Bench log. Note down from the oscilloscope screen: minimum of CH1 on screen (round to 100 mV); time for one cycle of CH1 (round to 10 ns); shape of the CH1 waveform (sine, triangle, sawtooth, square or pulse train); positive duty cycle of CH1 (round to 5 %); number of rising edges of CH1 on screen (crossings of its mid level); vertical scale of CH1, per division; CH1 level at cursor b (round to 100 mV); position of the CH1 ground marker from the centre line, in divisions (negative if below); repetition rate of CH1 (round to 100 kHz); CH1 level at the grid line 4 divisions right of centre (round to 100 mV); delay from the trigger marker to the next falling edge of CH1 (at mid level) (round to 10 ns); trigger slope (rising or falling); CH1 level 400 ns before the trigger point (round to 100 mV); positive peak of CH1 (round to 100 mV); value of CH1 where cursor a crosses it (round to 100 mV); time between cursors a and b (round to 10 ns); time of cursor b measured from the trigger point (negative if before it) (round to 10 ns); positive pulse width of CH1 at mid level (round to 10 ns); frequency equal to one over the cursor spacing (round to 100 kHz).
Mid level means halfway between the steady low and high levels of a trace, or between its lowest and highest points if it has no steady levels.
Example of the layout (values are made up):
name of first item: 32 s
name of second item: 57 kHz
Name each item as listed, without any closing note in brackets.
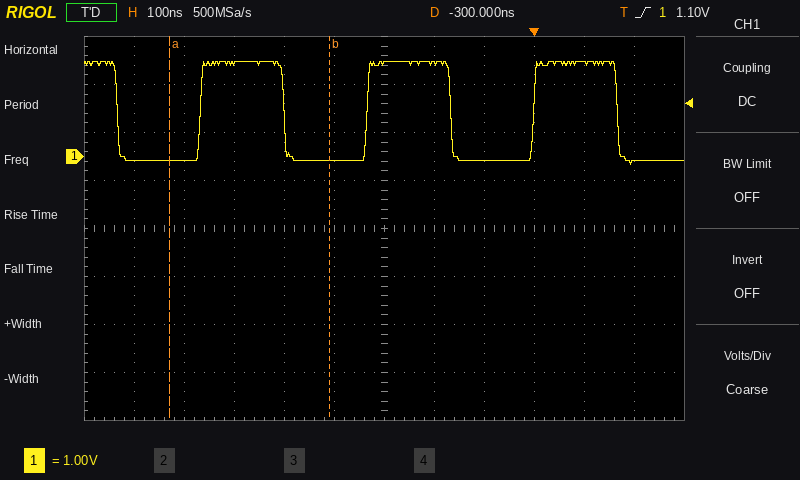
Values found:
minimum of CH1 on screen: -200 mV
time for one cycle of CH1: 330 ns
shape of the CH1 waveform: square
positive duty cycle of CH1: 50 %
number of rising edges of CH1 on screen: 3
vertical scale of CH1, per division: 1 V
CH1 level at cursor b: -100 mV
position of the CH1 ground marker from the centre line, in divisions: +1.5 div
repetition rate of CH1: 3.0 MHz
CH1 level at the grid line 4 divisions right of centre: 1.9 V
delay from the trigger marker to the next falling edge of CH1 (at mid level): 170 ns
trigger slope: rising
CH1 level 400 ns before the trigger point: -100 mV
positive peak of CH1: 2.0 V
value of CH1 where cursor a crosses it: -100 mV
time between cursors a and b: 320 ns
time of cursor b measured from the trigger point (negative if before it): -410 ns
positive pulse width of CH1 at mid level: 170 ns
frequency equal to one over the cursor spacing: 3.1 MHz
